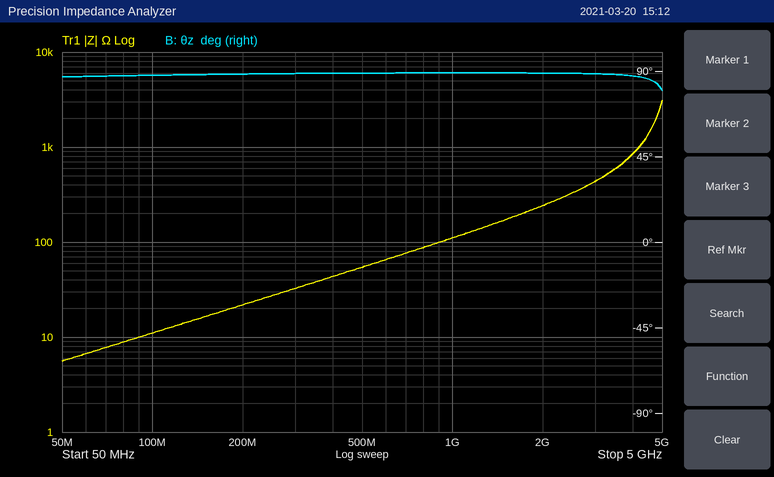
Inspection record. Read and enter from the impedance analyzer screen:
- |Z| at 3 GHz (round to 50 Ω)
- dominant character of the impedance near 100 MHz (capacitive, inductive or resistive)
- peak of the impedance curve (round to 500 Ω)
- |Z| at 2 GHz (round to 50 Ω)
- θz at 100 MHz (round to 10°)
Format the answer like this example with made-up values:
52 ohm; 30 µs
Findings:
450 Ω; inductive; 3.0 kΩ; 250 Ω; 90°
